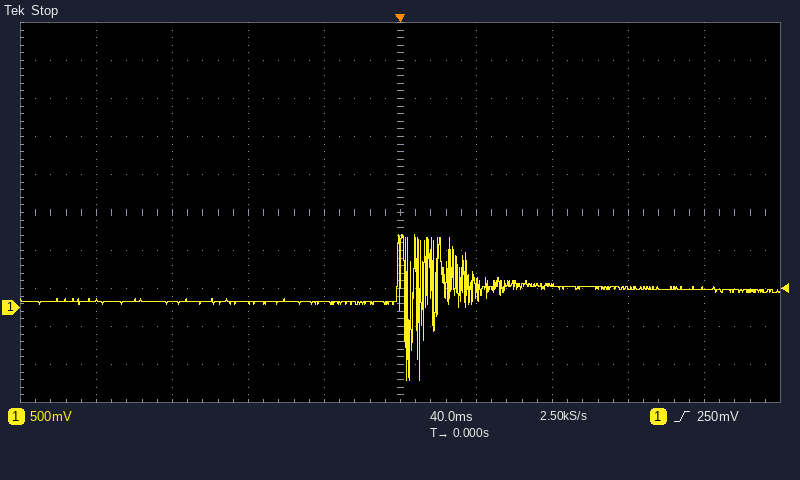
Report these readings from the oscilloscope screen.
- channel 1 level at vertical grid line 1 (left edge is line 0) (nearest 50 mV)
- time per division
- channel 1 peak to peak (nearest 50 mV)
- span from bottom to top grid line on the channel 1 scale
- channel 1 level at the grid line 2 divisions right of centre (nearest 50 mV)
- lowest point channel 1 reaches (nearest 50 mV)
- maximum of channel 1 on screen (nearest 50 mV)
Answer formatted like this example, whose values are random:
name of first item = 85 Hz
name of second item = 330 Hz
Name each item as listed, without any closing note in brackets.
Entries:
channel 1 level at vertical grid line 1 (left edge is line 0) = 100 mV
time per division = 40 ms
channel 1 peak to peak = 1.90 V
span from bottom to top grid line on the channel 1 scale = 5 V
channel 1 level at the grid line 2 divisions right of centre = 300 mV
lowest point channel 1 reaches = -950 mV
maximum of channel 1 on screen = 950 mV
